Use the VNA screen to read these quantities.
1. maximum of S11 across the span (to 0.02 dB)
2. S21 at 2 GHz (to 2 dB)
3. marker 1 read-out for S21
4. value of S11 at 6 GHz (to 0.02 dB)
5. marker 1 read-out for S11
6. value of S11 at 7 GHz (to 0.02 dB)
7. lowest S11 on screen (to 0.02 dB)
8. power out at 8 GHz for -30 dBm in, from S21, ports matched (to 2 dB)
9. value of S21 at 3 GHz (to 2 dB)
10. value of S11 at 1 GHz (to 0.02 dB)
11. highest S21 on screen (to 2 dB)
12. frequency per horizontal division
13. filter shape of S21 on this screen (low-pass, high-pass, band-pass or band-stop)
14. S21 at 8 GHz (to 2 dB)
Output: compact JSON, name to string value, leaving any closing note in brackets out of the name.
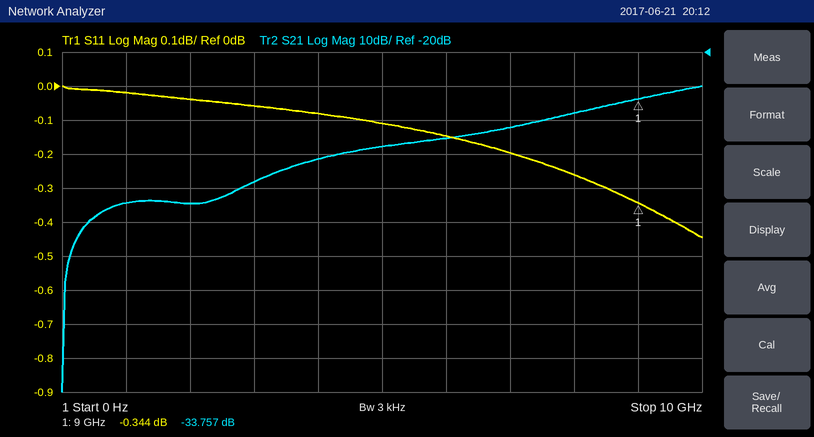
{"maximum of S11 across the span": "0.00 dB", "S21 at 2 GHz": "-64 dB", "marker 1 read-out for S21": "-33.757 dB", "value of S11 at 6 GHz": "-0.14 dB", "marker 1 read-out for S11": "-0.344 dB", "value of S11 at 7 GHz": "-0.20 dB", "lowest S11 on screen": "-0.44 dB", "power out at 8 GHz for -30 dBm in, from S21, ports matched": "-68 dBm", "value of S21 at 3 GHz": "-58 dB", "value of S11 at 1 GHz": "-0.02 dB", "highest S21 on screen": "-30 dB", "frequency per horizontal division": "1 GHz", "filter shape of S21 on this screen": "high-pass", "S21 at 8 GHz": "-38 dB"}
